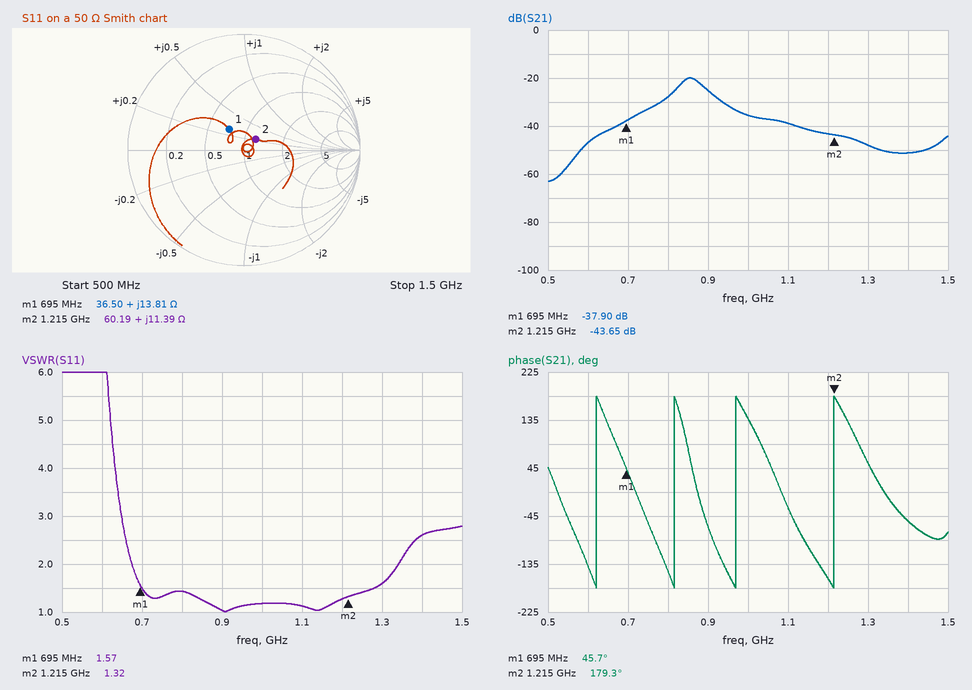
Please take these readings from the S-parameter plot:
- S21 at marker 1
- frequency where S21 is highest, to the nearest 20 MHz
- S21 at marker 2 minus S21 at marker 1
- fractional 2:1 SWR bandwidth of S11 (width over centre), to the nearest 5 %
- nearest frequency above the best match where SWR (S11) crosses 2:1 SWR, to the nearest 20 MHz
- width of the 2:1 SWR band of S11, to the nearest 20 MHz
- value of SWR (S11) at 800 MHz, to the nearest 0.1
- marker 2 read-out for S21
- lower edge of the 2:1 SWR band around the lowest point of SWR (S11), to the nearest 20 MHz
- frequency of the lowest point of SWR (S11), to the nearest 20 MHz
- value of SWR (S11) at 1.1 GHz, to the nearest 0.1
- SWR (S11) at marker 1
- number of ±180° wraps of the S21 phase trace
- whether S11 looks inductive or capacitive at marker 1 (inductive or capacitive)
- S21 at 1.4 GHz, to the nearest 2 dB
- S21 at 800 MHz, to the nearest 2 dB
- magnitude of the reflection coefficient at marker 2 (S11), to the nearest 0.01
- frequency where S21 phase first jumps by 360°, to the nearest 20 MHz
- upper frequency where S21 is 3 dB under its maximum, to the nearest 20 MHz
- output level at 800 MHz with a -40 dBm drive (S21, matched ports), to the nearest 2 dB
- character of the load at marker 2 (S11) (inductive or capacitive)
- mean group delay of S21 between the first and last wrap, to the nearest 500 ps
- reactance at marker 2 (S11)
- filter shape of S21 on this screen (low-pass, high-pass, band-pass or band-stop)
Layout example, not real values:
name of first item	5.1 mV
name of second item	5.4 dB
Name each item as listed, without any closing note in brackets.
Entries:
S21 at marker 1	-37.90 dB
frequency where S21 is highest, to the nearest 20 MHz	860 MHz
S21 at marker 2 minus S21 at marker 1	-5.75 dB
fractional 2:1 SWR bandwidth of S11 (width over centre), to the nearest 5 %	65 %
nearest frequency above the best match where SWR (S11) crosses 2:1 SWR, to the nearest 20 MHz	1.34 GHz
width of the 2:1 SWR band of S11, to the nearest 20 MHz	660 MHz
value of SWR (S11) at 800 MHz, to the nearest 0.1	1.4
marker 2 read-out for S21	-43.65 dB
lower edge of the 2:1 SWR band around the lowest point of SWR (S11), to the nearest 20 MHz	680 MHz
frequency of the lowest point of SWR (S11), to the nearest 20 MHz	900 MHz
value of SWR (S11) at 1.1 GHz, to the nearest 0.1	1.1
SWR (S11) at marker 1	1.57
number of ±180° wraps of the S21 phase trace	4
whether S11 looks inductive or capacitive at marker 1	inductive
S21 at 1.4 GHz, to the nearest 2 dB	-52 dB
S21 at 800 MHz, to the nearest 2 dB	-28 dB
magnitude of the reflection coefficient at marker 2 (S11), to the nearest 0.01	0.14
frequency where S21 phase first jumps by 360°, to the nearest 20 MHz	620 MHz
upper frequency where S21 is 3 dB under its maximum, to the nearest 20 MHz	880 MHz
output level at 800 MHz with a -40 dBm drive (S21, matched ports), to the nearest 2 dB	-68 dBm
character of the load at marker 2 (S11)	inductive
mean group delay of S21 between the first and last wrap, to the nearest 500 ps	5.0 ns
reactance at marker 2	+11.39 Ω
filter shape of S21 on this screen	band-pass
